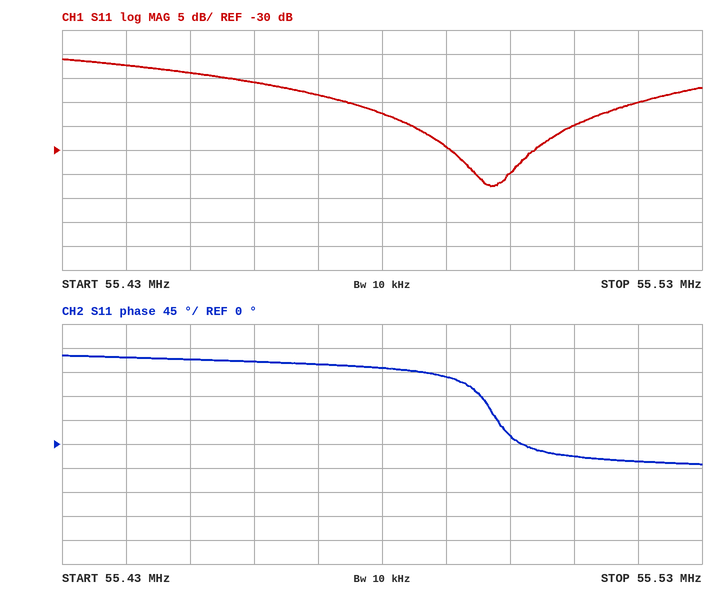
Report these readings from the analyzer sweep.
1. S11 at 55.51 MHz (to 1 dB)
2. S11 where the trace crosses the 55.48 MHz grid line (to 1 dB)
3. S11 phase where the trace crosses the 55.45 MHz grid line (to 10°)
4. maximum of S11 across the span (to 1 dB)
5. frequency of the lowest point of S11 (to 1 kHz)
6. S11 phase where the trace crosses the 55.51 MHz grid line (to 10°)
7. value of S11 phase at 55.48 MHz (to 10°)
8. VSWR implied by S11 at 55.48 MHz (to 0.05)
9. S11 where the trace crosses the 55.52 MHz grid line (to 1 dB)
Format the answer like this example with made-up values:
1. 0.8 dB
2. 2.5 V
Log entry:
1. -25 dB
2. -22 dB
3. 160°
4. -11 dB
5. 55.497 MHz
6. -20°
7. 140°
8. 1.15
9. -20 dB
